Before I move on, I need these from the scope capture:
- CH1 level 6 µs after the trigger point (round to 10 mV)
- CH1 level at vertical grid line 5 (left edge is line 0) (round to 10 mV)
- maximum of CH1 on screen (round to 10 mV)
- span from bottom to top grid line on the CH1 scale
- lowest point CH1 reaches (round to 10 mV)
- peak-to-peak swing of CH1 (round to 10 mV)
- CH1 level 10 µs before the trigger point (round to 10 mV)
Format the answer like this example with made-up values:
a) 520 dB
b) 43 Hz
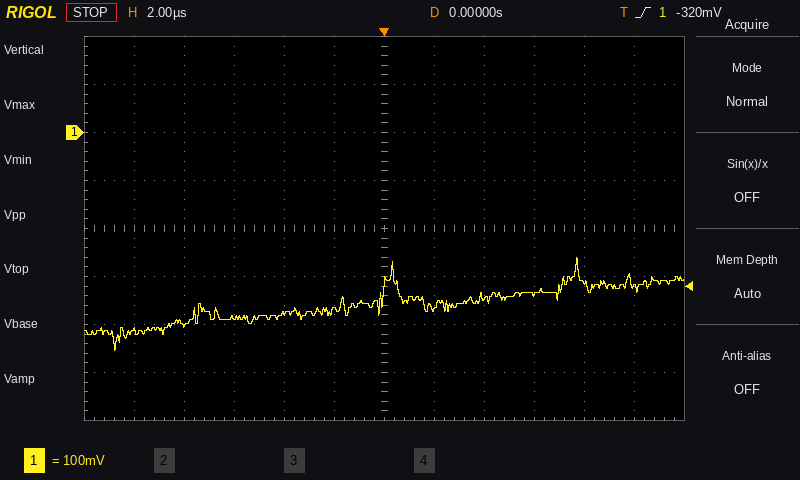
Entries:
a) -340 mV
b) -370 mV
c) -260 mV
d) 800 mV
e) -450 mV
f) 190 mV
g) -410 mV
